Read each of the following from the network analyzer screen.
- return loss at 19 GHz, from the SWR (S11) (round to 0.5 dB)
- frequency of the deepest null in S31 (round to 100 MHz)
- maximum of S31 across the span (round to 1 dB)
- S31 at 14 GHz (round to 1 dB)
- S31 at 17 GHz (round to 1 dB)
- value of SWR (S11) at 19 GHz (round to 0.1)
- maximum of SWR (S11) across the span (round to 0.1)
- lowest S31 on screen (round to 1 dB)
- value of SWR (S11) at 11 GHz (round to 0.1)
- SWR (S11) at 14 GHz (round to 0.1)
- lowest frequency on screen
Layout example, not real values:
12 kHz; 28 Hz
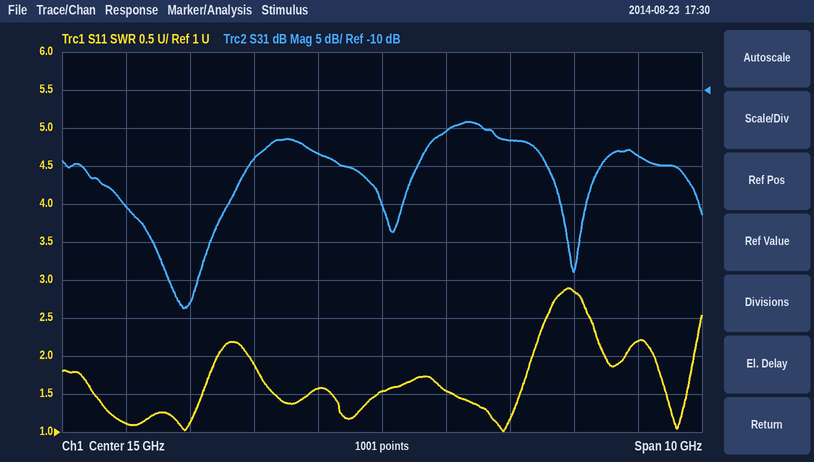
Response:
8.5 dB; 11.9 GHz; -14 dB; -18 dB; -17 dB; 2.2; 2.9; -39 dB; 1.1; 1.6; 10 GHz
